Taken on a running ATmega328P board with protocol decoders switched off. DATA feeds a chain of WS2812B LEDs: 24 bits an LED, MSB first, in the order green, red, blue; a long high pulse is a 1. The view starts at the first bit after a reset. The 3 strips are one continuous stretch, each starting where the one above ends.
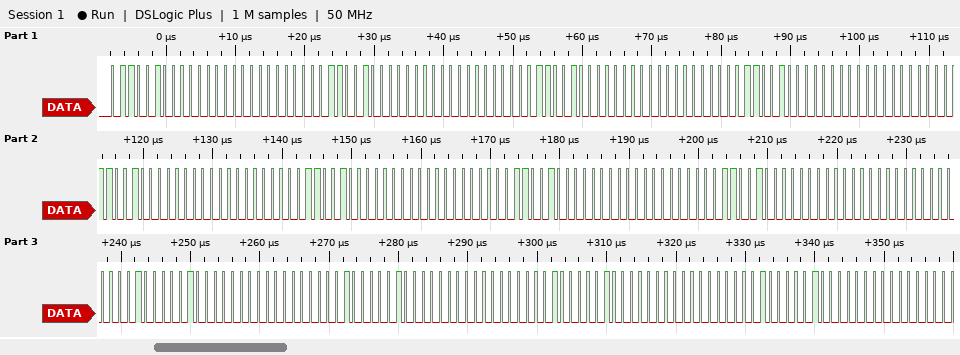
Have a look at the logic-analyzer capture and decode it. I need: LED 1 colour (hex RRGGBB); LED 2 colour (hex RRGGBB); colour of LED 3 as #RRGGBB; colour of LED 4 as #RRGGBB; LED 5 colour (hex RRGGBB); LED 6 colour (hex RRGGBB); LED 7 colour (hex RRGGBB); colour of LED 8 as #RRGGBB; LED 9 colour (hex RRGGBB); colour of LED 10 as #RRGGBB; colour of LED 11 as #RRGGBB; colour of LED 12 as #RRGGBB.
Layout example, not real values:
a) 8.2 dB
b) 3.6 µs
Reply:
a) #006400
b) #006400
c) #006400
d) #006400
e) #006400
f) #006400
g) #006400
h) #006400
i) #820000
j) #820000
k) #820000
l) #820000
